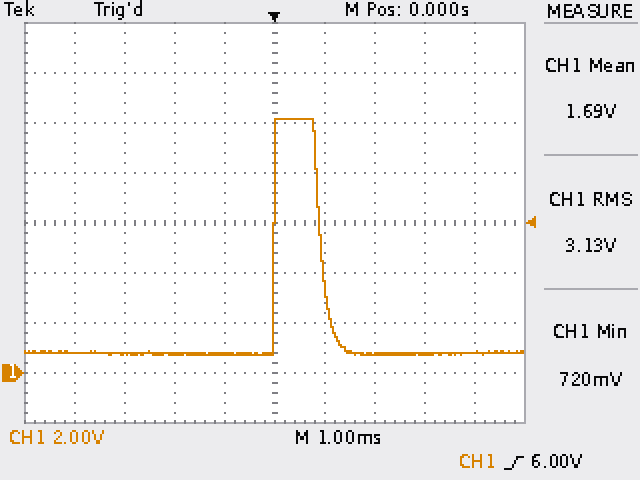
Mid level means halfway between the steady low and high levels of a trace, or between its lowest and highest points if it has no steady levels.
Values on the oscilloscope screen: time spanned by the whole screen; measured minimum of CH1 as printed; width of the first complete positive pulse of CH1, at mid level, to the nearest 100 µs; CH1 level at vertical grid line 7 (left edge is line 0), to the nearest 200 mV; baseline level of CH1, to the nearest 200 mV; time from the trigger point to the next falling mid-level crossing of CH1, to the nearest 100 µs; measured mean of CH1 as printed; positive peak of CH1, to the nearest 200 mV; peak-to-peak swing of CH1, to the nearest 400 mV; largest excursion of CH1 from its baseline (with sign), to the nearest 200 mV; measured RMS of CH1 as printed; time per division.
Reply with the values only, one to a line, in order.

10 ms
720 mV
900 µs
800 mV
800 mV
900 µs
1.69 V
10.2 V
9.6 V
+9.4 V
3.13 V
1 ms
